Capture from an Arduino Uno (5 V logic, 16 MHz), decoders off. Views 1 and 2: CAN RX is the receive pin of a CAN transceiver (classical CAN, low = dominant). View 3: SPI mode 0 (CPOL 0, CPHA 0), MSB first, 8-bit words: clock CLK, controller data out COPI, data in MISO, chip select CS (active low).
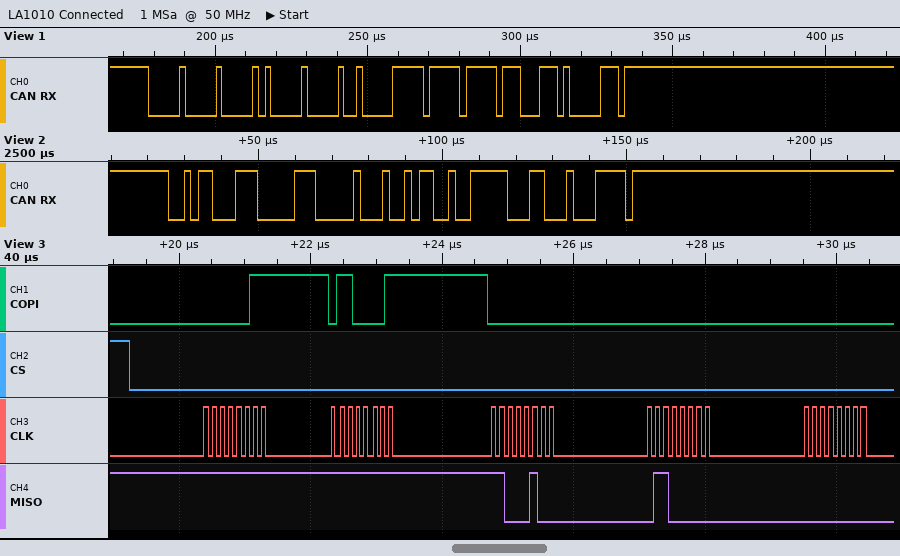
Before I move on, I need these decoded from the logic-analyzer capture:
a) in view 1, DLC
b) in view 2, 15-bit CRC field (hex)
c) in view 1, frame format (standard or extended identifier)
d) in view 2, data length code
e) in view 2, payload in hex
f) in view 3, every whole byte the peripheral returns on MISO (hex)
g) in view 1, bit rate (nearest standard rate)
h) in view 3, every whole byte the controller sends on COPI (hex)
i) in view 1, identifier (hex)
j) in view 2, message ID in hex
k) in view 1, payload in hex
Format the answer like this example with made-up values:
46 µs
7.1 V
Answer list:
4
0x4C47
standard
3
00 96 4F
FF FF C4 60 00
500 kbit/s
03 61 00 00 00
0x000
0x2C7
00 20 FF FF
